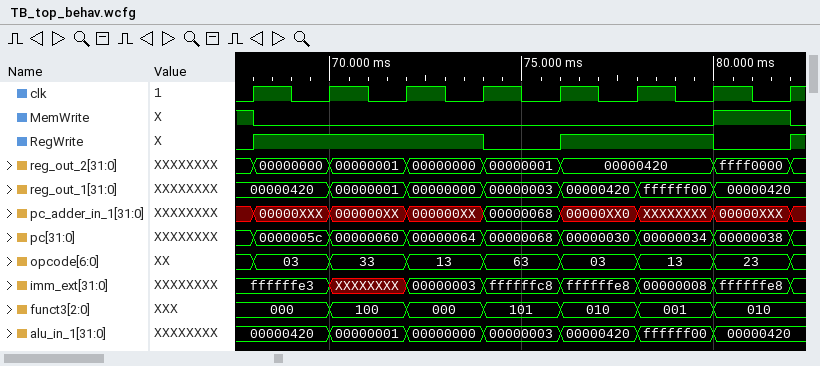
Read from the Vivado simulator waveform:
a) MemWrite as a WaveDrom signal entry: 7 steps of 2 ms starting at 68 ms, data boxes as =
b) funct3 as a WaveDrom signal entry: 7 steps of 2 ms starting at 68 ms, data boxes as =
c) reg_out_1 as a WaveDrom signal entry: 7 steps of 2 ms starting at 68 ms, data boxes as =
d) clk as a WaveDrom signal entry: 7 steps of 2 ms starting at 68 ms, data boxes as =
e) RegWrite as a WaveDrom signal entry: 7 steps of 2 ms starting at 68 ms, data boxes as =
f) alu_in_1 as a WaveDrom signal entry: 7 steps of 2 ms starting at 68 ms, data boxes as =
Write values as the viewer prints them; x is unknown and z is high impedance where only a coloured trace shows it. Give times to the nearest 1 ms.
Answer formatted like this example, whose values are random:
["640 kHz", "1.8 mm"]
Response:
["{name: 'MemWrite', wave: '0.....1'}", "{name: 'funct3', wave: '=======', data: '000 100 000 101 010 001 010'}", "{name: 'reg_out_1', wave: '=======', data: '00000420 00000001 00000000 00000003 00000420 ffffff00 00000420'}", "{name: 'clk', wave: 'p......'}", "{name: 'RegWrite', wave: '1..01.0'}", "{name: 'alu_in_1', wave: '=======', data: '00000420 00000001 00000000 00000003 00000420 ffffff00 00000420'}"]
